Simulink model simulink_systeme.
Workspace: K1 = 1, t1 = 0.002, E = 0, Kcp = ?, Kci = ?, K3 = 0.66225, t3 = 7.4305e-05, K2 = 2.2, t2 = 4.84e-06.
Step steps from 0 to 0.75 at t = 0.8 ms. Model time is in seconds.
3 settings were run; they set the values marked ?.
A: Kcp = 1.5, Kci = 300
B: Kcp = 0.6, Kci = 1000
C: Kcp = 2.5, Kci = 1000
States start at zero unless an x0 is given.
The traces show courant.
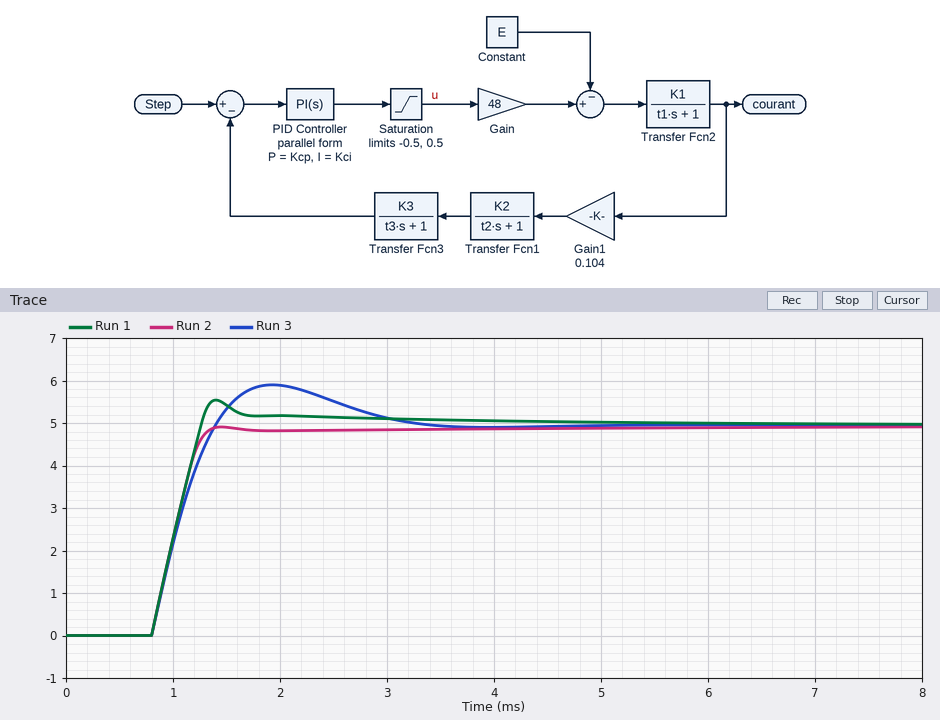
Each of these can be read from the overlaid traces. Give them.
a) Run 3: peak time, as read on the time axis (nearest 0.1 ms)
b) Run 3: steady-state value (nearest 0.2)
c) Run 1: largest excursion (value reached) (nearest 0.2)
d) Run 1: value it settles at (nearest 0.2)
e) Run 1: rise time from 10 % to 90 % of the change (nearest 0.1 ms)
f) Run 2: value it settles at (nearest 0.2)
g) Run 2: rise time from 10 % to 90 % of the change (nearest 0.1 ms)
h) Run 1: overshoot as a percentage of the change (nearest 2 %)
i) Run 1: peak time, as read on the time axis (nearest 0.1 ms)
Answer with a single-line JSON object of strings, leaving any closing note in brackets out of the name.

{"Run 3: peak time, as read on the time axis": "1.9 ms", "Run 3: steady-state value": "5.0", "Run 1: largest excursion (value reached)": "5.6", "Run 1: value it settles at": "5.0", "Run 1: rise time from 10 % to 90 % of the change": "0.4 ms", "Run 2: value it settles at": "5.0", "Run 2: rise time from 10 % to 90 % of the change": "0.4 ms", "Run 1: overshoot as a percentage of the change": "12 %", "Run 1: peak time, as read on the time axis": "1.4 ms"}
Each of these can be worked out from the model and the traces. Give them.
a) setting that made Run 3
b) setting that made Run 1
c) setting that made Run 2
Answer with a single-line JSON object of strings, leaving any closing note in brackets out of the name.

{"setting that made Run 3": "B", "setting that made Run 1": "C", "setting that made Run 2": "A"}
